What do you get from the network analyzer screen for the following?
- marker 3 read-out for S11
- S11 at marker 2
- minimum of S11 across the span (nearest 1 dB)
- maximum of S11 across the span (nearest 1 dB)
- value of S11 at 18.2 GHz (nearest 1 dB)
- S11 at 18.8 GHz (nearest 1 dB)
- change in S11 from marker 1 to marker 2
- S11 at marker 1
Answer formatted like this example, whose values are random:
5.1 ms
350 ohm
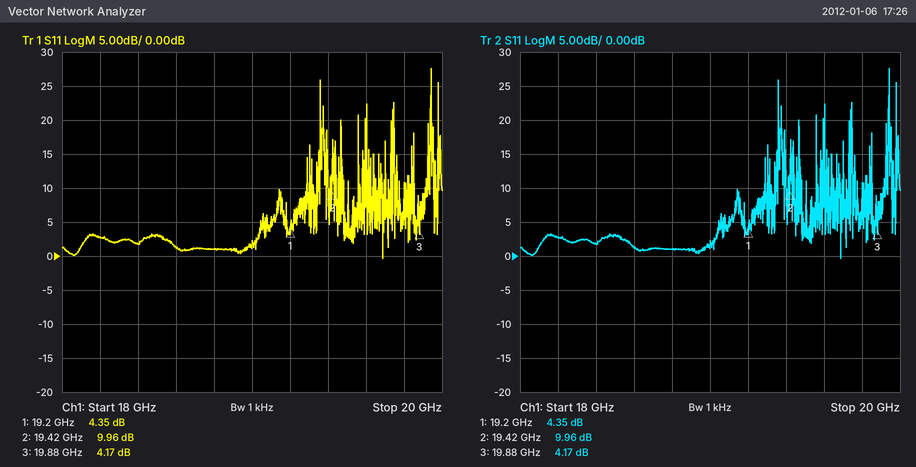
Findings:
4.17 dB
9.96 dB
0 dB
28 dB
3 dB
1 dB
5.61 dB
4.35 dB
